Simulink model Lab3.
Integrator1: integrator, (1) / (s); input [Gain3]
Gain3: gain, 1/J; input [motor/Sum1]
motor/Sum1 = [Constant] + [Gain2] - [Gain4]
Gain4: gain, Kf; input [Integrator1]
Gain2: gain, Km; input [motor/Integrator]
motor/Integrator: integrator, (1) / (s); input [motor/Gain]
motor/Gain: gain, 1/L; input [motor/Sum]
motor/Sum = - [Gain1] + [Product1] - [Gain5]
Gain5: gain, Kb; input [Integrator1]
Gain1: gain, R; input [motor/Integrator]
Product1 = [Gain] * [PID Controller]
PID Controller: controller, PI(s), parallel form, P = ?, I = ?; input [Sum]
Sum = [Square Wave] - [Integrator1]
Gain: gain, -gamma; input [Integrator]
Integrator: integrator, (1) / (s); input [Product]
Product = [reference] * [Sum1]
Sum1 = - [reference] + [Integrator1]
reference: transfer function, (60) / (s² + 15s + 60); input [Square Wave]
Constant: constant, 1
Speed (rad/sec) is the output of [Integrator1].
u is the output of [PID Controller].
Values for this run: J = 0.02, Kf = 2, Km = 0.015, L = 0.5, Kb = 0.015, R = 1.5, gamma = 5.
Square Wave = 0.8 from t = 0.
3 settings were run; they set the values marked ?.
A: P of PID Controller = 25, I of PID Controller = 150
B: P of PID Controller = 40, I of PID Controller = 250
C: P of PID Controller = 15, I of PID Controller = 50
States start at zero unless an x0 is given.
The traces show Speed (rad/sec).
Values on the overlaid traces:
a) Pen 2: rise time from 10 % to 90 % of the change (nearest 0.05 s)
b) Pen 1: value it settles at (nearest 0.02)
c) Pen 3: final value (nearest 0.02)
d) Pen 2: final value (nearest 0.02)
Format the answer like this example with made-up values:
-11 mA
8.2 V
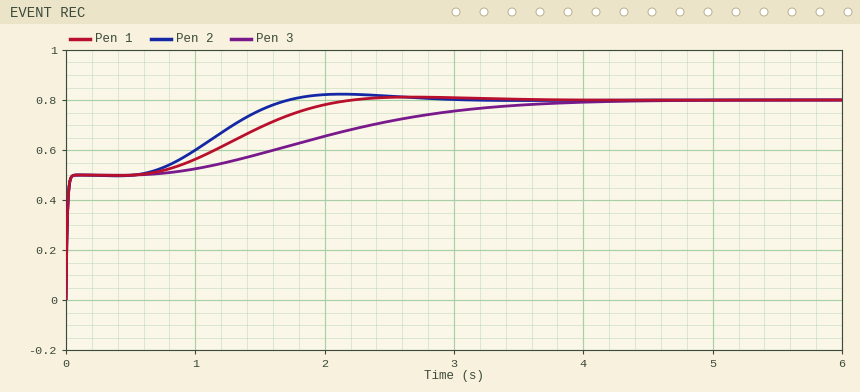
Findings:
1.35 s
0.80
0.80
0.80
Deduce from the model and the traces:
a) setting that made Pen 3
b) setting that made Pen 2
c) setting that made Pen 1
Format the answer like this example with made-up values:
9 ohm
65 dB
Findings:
C
B
A
